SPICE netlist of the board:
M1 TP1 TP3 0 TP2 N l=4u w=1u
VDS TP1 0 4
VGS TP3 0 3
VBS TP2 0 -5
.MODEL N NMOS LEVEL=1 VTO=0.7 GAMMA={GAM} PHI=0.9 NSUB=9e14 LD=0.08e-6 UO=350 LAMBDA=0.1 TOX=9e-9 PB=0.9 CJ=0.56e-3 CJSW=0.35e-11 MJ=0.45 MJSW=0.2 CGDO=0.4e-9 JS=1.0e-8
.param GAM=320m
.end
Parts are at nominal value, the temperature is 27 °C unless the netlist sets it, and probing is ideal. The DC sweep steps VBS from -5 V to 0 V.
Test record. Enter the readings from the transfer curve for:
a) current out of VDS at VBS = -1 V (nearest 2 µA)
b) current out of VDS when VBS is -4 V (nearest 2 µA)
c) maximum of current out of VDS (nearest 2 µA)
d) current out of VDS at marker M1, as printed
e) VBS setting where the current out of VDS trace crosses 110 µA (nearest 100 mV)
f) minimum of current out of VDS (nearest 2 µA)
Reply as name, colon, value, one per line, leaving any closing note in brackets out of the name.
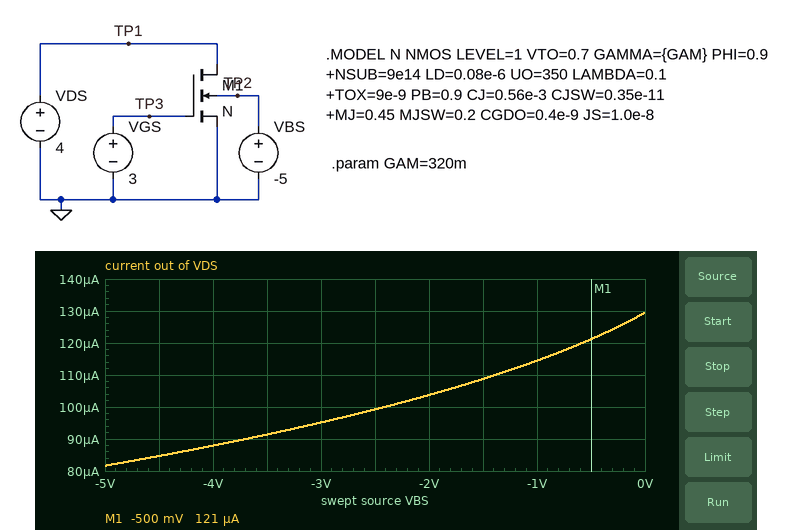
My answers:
current out of VDS at VBS = -1 V: 114 µA
current out of VDS when VBS is -4 V: 88 µA
maximum of current out of VDS: 130 µA
current out of VDS at marker M1, as printed: 121 µA
VBS setting where the current out of VDS trace crosses 110 µA: -1.4 V
minimum of current out of VDS: 82 µA
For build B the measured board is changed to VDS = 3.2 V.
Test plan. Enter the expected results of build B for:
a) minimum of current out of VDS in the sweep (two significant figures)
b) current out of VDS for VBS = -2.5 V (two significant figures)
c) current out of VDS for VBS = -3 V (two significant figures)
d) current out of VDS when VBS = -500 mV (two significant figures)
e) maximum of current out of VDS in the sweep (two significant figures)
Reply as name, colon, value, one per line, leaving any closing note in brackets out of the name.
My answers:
minimum of current out of VDS in the sweep: 77 µA
current out of VDS for VBS = -2.5 V: 94 µA
current out of VDS for VBS = -3 V: 90 µA
current out of VDS when VBS = -500 mV: 110 µA
maximum of current out of VDS in the sweep: 120 µA
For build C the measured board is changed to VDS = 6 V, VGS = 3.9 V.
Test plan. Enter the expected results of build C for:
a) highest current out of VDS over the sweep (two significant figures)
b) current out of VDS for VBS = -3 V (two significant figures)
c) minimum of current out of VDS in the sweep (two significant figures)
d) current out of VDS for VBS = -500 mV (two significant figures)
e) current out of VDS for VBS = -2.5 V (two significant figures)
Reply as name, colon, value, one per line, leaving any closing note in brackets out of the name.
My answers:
highest current out of VDS over the sweep: 290 µA
current out of VDS for VBS = -3 V: 230 µA
minimum of current out of VDS in the sweep: 210 µA
current out of VDS for VBS = -500 mV: 270 µA
current out of VDS for VBS = -2.5 V: 240 µA
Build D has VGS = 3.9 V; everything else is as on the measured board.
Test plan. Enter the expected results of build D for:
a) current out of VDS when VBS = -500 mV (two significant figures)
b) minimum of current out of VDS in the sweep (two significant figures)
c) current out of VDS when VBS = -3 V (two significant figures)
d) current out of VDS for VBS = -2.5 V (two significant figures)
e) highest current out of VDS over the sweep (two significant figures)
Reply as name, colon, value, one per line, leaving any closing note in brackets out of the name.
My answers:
current out of VDS when VBS = -500 mV: 240 µA
minimum of current out of VDS in the sweep: 180 µA
current out of VDS when VBS = -3 V: 200 µA
current out of VDS for VBS = -2.5 V: 210 µA
highest current out of VDS over the sweep: 250 µA
